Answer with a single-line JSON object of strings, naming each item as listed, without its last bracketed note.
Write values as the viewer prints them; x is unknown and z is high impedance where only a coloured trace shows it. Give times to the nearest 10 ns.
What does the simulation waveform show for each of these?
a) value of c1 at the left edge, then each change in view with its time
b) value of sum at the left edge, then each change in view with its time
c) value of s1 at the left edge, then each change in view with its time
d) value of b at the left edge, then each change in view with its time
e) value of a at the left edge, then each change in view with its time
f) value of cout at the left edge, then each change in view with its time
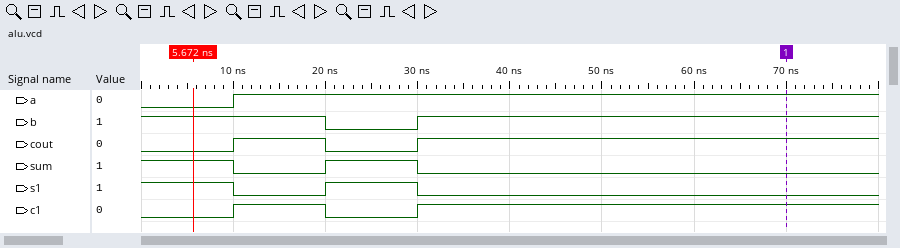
{"value of c1 at the left edge, then each change in view with its time": "0, 1 at 10 ns, 0 at 20 ns, 1 at 30 ns", "value of sum at the left edge, then each change in view with its time": "1, 0 at 10 ns, 1 at 20 ns, 0 at 30 ns", "value of s1 at the left edge, then each change in view with its time": "1, 0 at 10 ns, 1 at 20 ns, 0 at 30 ns", "value of b at the left edge, then each change in view with its time": "1, 0 at 20 ns, 1 at 30 ns", "value of a at the left edge, then each change in view with its time": "0, 1 at 10 ns", "value of cout at the left edge, then each change in view with its time": "0, 1 at 10 ns, 0 at 20 ns, 1 at 30 ns"}
